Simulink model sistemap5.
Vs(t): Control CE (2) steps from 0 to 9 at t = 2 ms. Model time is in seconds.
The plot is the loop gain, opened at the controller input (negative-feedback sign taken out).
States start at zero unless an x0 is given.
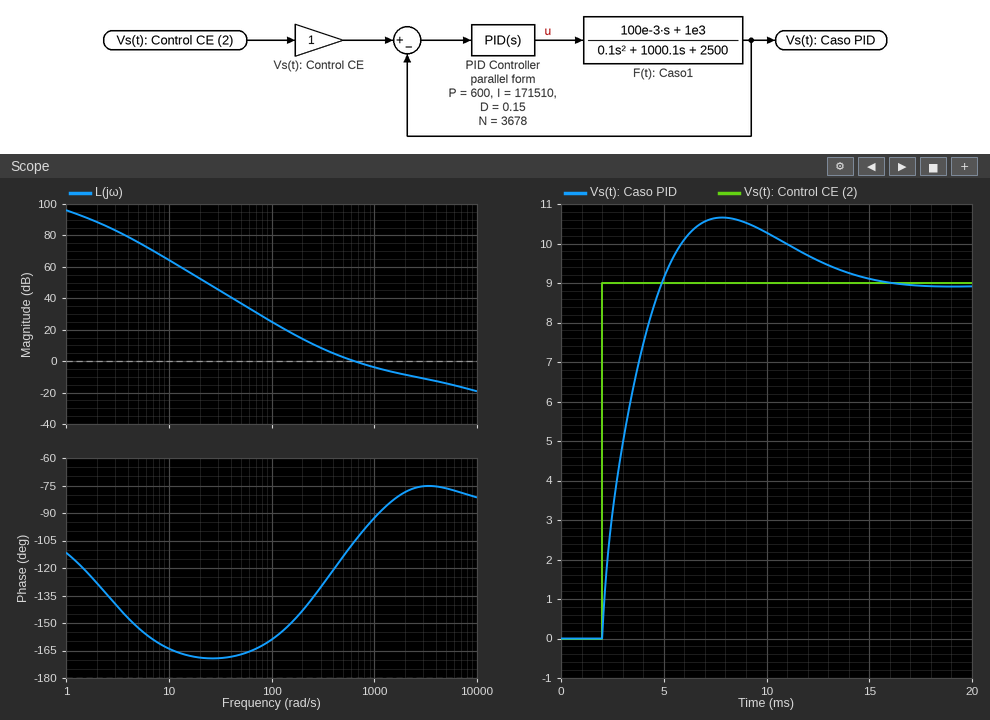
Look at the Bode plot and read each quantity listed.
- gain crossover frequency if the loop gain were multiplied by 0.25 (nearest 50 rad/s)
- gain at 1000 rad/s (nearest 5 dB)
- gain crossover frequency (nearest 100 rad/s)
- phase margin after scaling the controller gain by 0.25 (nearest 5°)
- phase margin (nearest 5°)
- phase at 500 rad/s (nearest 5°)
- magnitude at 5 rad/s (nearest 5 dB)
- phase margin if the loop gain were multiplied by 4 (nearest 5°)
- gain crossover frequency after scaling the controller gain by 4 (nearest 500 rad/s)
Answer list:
250 rad/s
-5 dB
600 rad/s
40°
75°
-115°
75 dB
105°
3500 rad/s
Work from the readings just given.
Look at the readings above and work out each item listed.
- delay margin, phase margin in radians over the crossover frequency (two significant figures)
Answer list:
0.0022 s
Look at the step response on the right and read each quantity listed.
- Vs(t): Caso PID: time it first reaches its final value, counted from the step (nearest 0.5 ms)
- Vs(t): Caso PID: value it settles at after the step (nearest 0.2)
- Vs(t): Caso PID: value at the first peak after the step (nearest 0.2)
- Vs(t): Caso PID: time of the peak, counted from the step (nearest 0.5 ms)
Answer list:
3.0 ms
9.0
10.6
6.0 ms
